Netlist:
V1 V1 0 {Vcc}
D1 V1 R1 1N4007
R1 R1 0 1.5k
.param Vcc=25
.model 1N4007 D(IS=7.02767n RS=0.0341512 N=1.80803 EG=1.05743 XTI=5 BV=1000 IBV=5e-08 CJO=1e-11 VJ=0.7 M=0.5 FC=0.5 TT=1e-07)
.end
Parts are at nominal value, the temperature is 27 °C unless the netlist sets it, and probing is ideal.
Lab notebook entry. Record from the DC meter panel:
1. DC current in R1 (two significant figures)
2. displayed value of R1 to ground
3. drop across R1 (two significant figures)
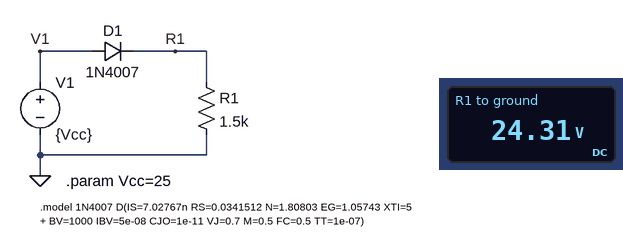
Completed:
16 mA
24.31 V
24 V
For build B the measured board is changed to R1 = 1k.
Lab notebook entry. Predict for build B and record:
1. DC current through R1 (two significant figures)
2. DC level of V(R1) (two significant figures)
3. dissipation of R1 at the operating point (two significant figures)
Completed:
24 mA
24 V
590 mW
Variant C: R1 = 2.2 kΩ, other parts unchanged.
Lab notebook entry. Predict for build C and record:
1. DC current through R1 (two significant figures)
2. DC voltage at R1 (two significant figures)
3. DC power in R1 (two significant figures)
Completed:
11 mA
24 V
270 mW
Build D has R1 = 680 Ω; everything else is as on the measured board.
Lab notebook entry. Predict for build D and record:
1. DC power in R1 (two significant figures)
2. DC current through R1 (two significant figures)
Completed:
870 mW
36 mA
